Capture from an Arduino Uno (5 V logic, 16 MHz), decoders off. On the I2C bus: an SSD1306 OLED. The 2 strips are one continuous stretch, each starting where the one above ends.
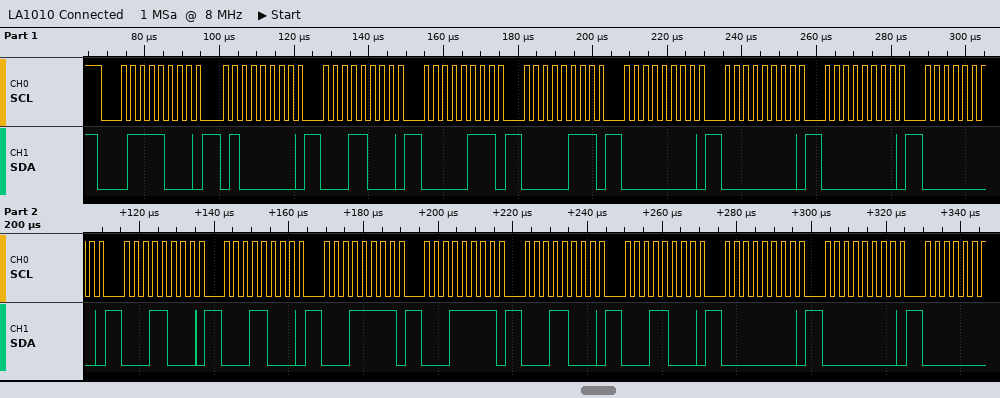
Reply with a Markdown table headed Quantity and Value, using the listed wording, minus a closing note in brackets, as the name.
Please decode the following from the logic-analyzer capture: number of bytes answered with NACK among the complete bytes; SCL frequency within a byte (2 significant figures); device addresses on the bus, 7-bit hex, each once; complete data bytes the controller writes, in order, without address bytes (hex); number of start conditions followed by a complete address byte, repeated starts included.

| Quantity | Value |
|---|---|
| number of bytes answered with NACK among the complete bytes | 0 |
| SCL frequency within a byte | 400 kHz |
| device addresses on the bus, 7-bit hex, each once | 0x3C |
| complete data bytes the controller writes, in order, without address bytes | 40 18 07 07 00 00 00 00 18 18 1F 1F 18 18 00 00 |
| number of start conditions followed by a complete address byte, repeated starts included | 1 |
